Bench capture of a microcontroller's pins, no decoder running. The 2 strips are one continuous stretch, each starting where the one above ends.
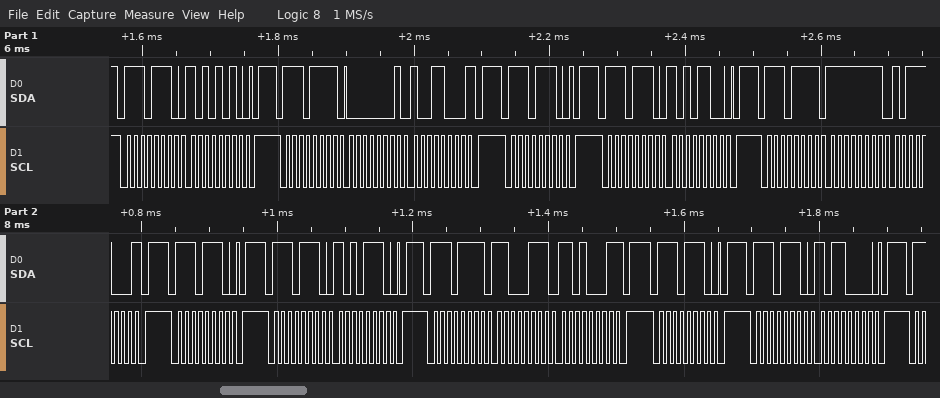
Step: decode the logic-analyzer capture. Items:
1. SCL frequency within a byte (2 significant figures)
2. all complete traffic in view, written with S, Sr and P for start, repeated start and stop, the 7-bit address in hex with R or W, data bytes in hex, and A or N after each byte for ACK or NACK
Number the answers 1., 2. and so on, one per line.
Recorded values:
1. 100 kHz
2. S 77W A AA A P S 77R A 01 A 98 N P S 77W A P S 77W A AC A P S 77R A FF A B8 N P S 77W A P S 77W A AE A P S 77R A C7 A D1 N P S 77W A P S 77W A B0 A P
